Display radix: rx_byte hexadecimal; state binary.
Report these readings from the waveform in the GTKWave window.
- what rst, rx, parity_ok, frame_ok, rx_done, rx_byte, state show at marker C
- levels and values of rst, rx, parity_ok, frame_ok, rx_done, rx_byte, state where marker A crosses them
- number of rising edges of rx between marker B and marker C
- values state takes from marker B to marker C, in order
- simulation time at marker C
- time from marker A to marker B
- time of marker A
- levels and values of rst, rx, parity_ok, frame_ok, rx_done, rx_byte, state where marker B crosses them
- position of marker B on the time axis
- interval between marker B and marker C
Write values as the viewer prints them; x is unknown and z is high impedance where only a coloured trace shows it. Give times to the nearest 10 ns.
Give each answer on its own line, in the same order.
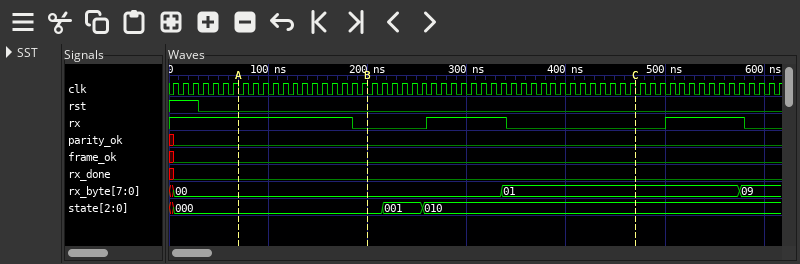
rst=0, rx=0, parity_ok=0, frame_ok=0, rx_done=0, rx_byte=01, state=010
rst=0, rx=1, parity_ok=0, frame_ok=0, rx_done=0, rx_byte=00, state=000
1
000, 001, 010
470 ns
130 ns
70 ns
rst=0, rx=0, parity_ok=0, frame_ok=0, rx_done=0, rx_byte=00, state=000
200 ns
270 ns
